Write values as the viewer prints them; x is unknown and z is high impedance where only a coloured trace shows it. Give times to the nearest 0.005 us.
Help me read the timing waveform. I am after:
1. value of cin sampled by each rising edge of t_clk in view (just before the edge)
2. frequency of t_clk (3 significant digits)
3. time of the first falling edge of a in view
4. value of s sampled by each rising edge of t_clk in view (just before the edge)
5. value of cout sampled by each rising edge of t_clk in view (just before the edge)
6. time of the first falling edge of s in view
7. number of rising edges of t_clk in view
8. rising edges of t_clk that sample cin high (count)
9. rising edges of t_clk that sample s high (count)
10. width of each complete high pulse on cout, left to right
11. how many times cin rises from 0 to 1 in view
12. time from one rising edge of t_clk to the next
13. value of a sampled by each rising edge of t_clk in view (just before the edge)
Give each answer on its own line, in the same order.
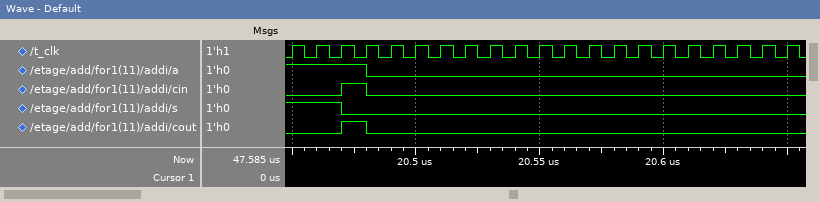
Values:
0 0 0 1 0 0 0 0 0 0 0 0 0 0 0 0 0 0 0 0 0
100 MHz
20.48 us
1 1 1 0 0 0 0 0 0 0 0 0 0 0 0 0 0 0 0 0 0
0 0 0 1 0 0 0 0 0 0 0 0 0 0 0 0 0 0 0 0 0
20.47 us
21
1
3
0.01 us
1
0.01 us
1 1 1 1 0 0 0 0 0 0 0 0 0 0 0 0 0 0 0 0 0
